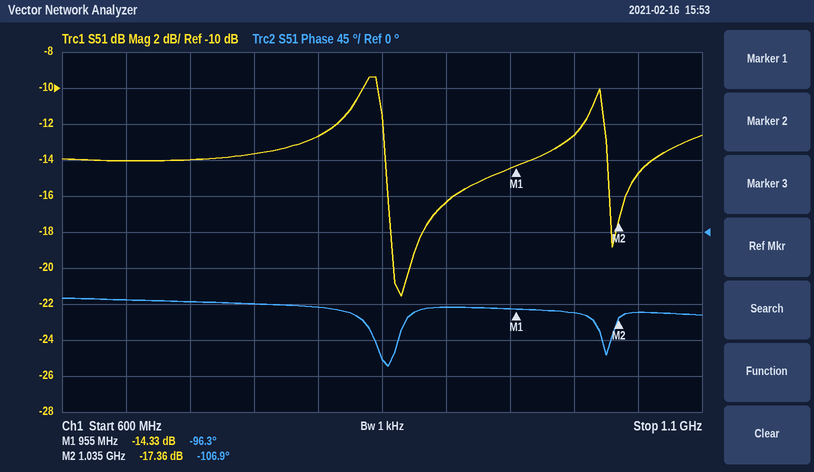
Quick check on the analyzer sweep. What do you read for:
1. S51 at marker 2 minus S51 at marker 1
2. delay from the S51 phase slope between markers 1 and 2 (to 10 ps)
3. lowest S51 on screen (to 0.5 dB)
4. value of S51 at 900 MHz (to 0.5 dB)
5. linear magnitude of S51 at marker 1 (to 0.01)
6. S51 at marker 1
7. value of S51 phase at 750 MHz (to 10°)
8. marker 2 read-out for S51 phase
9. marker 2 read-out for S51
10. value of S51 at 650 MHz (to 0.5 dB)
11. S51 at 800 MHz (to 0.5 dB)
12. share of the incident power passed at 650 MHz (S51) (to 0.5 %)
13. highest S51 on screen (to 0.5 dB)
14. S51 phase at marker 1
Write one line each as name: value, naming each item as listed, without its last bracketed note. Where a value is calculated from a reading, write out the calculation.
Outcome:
S51 at marker 2 minus S51 at marker 1: -17.36 − (-14.33) = -3.03 dB
delay from the S51 phase slope between markers 1 and 2: −(-106.9° − (-96.3°))/(360° × 80 MHz) ≈ 368 ps, so 370 ps to the nearest 10 ps
lowest S51 on screen: -21.5 dB
value of S51 at 900 MHz: -16.5 dB
linear magnitude of S51 at marker 1: 10^(-14.33/20) ≈ 0.19
S51 at marker 1: -14.33 dB
value of S51 phase at 750 MHz: -90°
marker 2 read-out for S51 phase: -106.9°
marker 2 read-out for S51: -17.36 dB
value of S51 at 650 MHz: -14.0 dB
S51 at 800 MHz: -12.5 dB
share of the incident power passed at 650 MHz (S51): 10^(-14/10) ≈ 4.0 %
highest S51 on screen: -9.5 dB
S51 phase at marker 1: -96.3°
